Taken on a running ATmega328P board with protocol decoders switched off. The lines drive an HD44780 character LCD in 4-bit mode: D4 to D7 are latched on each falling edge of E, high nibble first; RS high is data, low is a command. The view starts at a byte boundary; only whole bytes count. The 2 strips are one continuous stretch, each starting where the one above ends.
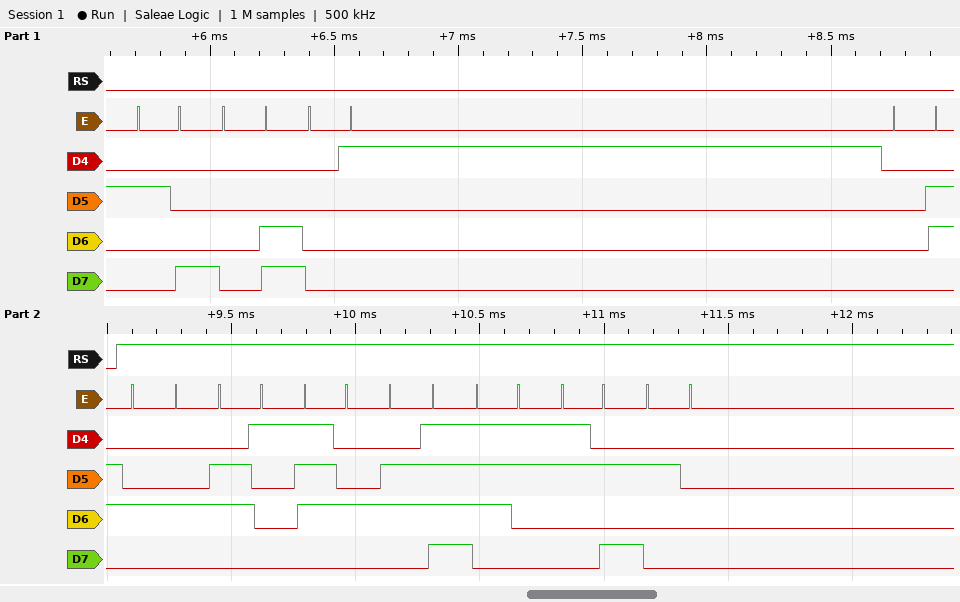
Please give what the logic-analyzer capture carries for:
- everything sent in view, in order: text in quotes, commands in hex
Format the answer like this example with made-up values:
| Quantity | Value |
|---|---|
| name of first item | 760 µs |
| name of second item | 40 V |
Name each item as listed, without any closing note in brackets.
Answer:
| Quantity | Value |
|---|---|
| everything sent in view, in order: text in quotes, commands in hex | 0x28 0x0C 0x01 0x06 "Datos: " |
